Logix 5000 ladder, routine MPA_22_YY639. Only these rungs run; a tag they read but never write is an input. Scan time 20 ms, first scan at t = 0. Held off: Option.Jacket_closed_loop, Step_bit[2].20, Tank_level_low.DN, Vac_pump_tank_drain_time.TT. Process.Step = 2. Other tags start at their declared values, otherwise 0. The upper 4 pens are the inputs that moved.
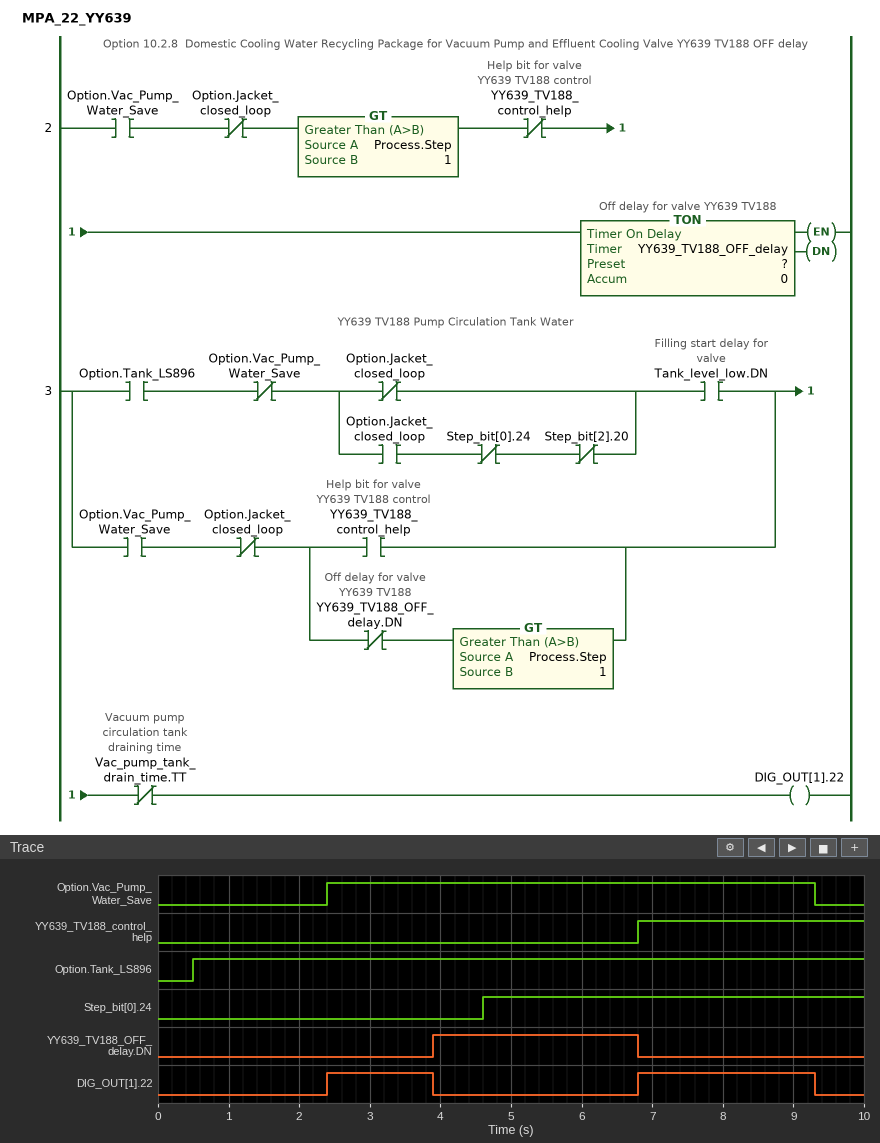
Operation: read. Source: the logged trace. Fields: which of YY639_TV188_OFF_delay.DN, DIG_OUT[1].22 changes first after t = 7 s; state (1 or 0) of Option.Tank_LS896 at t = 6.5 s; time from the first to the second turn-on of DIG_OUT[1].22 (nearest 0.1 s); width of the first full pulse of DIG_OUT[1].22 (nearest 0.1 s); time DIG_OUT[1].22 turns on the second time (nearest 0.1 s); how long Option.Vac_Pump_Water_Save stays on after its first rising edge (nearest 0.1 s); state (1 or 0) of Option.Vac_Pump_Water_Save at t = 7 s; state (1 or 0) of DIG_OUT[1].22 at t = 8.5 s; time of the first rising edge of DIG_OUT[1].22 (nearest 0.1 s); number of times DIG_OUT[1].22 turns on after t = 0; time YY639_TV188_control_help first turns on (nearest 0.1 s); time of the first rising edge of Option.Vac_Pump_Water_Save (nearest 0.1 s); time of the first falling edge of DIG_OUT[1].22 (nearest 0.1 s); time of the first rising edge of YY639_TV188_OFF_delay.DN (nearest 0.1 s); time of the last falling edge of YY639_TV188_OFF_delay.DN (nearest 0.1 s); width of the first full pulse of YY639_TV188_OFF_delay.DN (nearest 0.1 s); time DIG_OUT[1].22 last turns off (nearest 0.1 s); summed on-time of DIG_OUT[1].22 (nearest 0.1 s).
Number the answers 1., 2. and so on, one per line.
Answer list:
1. DIG_OUT[1].22
2. 1
3. 4.4 s
4. 1.5 s
5. 6.8 s
6. 6.9 s
7. 1
8. 1
9. 2.4 s
10. 2
11. 6.8 s
12. 2.4 s
13. 3.9 s
14. 3.9 s
15. 6.8 s
16. 2.9 s
17. 9.3 s
18. 4.0 s
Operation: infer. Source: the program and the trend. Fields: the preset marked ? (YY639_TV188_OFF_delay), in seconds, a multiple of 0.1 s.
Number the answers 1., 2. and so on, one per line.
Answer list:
1. 1.5 s
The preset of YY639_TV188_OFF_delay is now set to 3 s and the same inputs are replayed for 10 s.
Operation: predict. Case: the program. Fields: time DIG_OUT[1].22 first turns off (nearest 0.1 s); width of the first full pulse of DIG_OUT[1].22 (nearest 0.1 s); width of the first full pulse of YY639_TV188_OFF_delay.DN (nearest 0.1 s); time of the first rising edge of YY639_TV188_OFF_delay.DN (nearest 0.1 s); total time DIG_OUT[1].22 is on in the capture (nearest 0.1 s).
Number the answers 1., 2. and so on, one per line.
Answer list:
1. 5.4 s
2. 3.0 s
3. 1.4 s
4. 5.4 s
5. 5.5 s
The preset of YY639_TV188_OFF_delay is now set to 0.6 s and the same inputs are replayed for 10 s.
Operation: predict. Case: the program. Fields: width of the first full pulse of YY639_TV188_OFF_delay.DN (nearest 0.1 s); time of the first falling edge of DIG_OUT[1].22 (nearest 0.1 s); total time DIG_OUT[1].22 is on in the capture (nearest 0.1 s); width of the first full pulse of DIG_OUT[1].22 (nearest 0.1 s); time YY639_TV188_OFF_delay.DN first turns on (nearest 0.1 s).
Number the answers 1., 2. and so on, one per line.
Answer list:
1. 3.8 s
2. 3.0 s
3. 3.1 s
4. 0.6 s
5. 3.0 s
